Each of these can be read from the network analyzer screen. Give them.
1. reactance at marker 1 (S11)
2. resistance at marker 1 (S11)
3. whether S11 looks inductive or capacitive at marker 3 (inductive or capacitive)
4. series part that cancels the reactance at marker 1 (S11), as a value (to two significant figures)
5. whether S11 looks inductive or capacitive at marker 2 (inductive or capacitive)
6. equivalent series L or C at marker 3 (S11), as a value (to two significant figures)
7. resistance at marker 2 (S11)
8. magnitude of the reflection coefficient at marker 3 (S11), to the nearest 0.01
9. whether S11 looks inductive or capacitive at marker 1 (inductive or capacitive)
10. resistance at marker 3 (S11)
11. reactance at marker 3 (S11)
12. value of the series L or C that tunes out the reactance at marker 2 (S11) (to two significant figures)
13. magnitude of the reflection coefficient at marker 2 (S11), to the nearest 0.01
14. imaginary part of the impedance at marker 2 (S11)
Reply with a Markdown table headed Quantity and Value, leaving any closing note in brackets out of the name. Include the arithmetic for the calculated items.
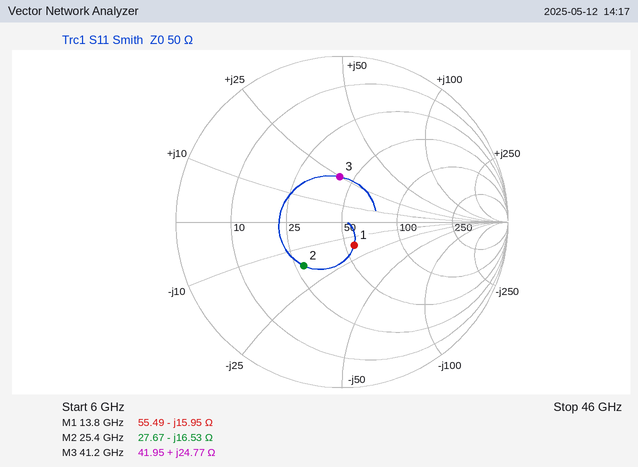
| Quantity | Value |
|---|---|
| reactance at marker 1 | -15.95 Ω |
| resistance at marker 1 | 55.49 Ω |
| whether S11 looks inductive or capacitive at marker 3 | inductive |
| series part that cancels the reactance at marker 1 (S11), as a value | L = 15.95 Ω/(2π × 13.8 GHz) ≈ 184 pH, so 180 pH to two significant figures |
| whether S11 looks inductive or capacitive at marker 2 | capacitive |
| equivalent series L or C at marker 3 (S11), as a value | L = 24.77 Ω/(2π × 41.2 GHz) ≈ 96 pH |
| resistance at marker 2 | 27.67 Ω |
| magnitude of the reflection coefficient at marker 3 (S11), to the nearest 0.01 | 0.27 |
| whether S11 looks inductive or capacitive at marker 1 | capacitive |
| resistance at marker 3 | 41.95 Ω |
| reactance at marker 3 | +24.77 Ω |
| value of the series L or C that tunes out the reactance at marker 2 (S11) | L = 16.53 Ω/(2π × 25.4 GHz) ≈ 104 pH, so 100 pH to two significant figures |
| magnitude of the reflection coefficient at marker 2 (S11), to the nearest 0.01 | 0.35 |
| imaginary part of the impedance at marker 2 | -16.53 Ω |
